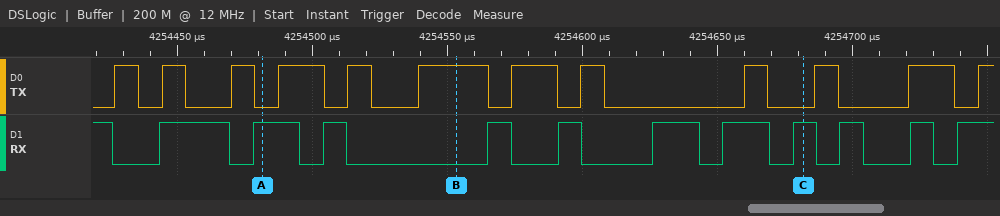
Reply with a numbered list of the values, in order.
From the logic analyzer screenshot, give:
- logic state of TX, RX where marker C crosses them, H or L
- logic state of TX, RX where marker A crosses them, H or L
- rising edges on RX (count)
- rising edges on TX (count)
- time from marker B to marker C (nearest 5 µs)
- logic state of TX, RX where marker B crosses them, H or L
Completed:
1. TX=L, RX=H
2. TX=L, RX=H
3. 11
4. 12
5. 130 µs
6. TX=H, RX=L
